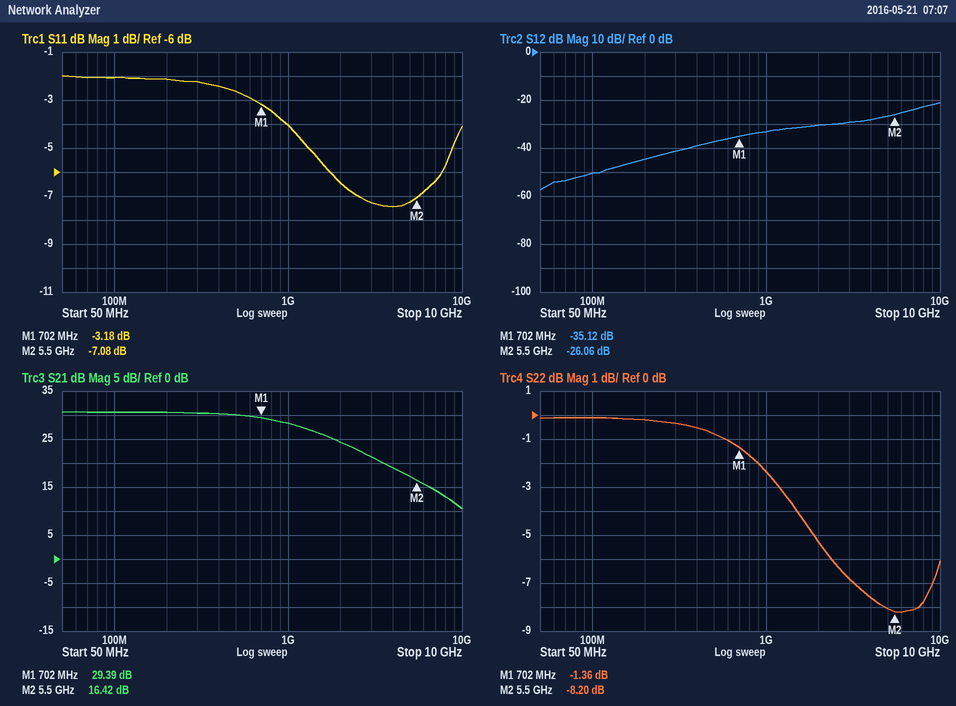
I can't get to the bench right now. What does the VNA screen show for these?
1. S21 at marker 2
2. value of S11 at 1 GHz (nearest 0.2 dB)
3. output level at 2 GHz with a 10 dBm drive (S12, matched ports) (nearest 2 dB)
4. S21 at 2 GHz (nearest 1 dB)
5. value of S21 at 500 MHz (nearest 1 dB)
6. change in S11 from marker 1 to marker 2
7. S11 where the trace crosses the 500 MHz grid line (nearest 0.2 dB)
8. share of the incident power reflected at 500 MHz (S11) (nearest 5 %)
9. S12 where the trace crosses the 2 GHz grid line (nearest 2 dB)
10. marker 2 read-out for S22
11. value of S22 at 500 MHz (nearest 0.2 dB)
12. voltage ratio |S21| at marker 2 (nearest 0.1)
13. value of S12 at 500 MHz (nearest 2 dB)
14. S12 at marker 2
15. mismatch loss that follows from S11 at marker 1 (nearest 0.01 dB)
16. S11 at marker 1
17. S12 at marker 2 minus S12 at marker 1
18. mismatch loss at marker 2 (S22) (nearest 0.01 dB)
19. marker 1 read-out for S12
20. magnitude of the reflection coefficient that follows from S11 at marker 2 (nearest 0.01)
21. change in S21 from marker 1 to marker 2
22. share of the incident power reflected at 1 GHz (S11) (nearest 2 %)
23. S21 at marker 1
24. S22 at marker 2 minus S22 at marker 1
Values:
16.42 dB
-4.0 dB
-20 dBm
24 dB
30 dB
-3.90 dB
-2.6 dB
55 %
-30 dB
-8.20 dB
-0.8 dB
6.6
-38 dB
-26.06 dB
2.85 dB
-3.18 dB
9.06 dB
0.71 dB
-35.12 dB
0.44
-12.97 dB
40 %
29.39 dB
-6.84 dB
